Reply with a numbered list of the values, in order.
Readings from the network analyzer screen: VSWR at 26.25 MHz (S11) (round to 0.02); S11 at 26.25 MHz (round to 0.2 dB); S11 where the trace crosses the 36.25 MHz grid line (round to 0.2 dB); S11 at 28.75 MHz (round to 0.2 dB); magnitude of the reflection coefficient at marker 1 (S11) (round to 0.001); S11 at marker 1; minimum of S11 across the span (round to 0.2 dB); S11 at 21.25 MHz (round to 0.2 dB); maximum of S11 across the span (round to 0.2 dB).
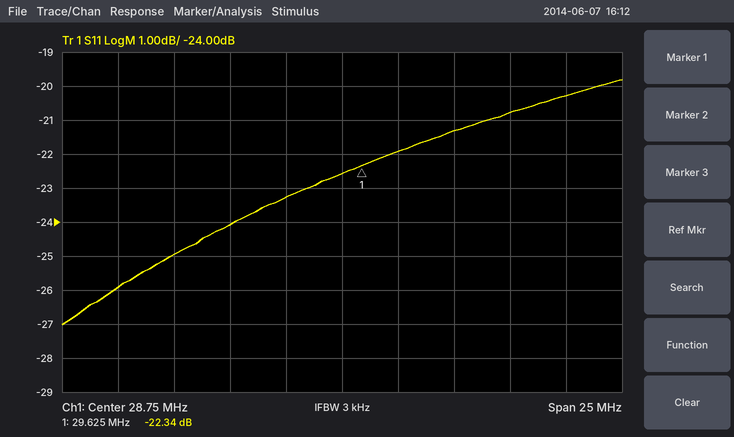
1. 1.14
2. -23.2 dB
3. -20.8 dB
4. -22.6 dB
5. 0.076
6. -22.34 dB
7. -27.0 dB
8. -25.0 dB
9. -19.8 dB
